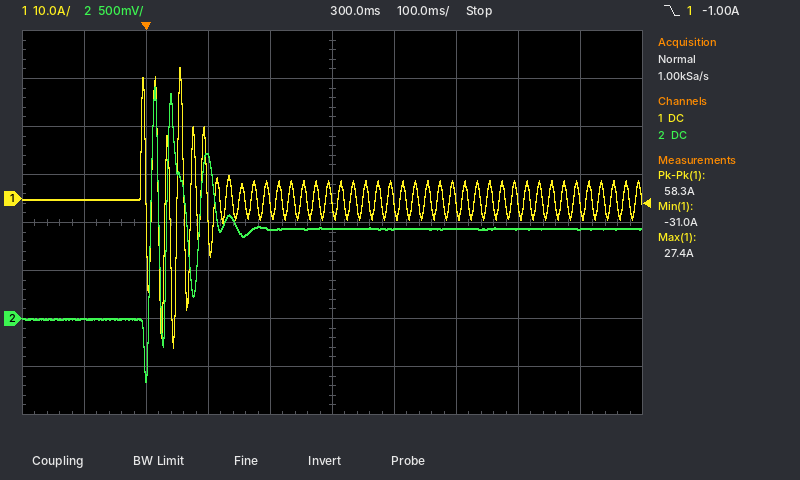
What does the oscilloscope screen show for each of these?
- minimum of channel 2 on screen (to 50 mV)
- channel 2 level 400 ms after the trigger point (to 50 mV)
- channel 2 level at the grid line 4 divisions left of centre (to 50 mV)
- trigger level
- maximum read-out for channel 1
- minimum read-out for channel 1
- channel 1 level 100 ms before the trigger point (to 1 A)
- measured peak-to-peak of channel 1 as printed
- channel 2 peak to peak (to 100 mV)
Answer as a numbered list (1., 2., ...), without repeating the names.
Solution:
1. -650 mV
2. 950 mV
3. 0 mV
4. -1.00 A
5. 27.4 A
6. -31.0 A
7. 0 A
8. 58.3 A
9. 3.10 V
